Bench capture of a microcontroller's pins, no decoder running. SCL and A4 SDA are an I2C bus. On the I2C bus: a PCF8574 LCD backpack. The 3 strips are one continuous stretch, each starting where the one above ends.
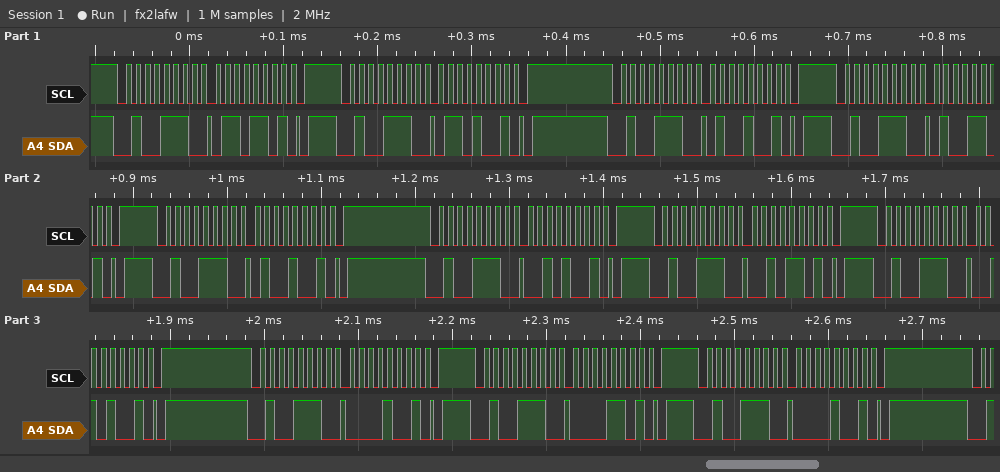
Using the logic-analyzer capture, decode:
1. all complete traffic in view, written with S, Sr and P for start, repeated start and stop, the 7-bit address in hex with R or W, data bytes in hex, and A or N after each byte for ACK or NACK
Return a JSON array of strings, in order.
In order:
["S 27W A 6D A P S 27W A 69 A P S 27W A 49 A P S 27W A 4D A P S 27W A 49 A P S 27W A 29 A P S 27W A 2D A P S 27W A 29 A P S 27W A 09 A P S 27W A 0D A P S 27W A 09 A P"]
